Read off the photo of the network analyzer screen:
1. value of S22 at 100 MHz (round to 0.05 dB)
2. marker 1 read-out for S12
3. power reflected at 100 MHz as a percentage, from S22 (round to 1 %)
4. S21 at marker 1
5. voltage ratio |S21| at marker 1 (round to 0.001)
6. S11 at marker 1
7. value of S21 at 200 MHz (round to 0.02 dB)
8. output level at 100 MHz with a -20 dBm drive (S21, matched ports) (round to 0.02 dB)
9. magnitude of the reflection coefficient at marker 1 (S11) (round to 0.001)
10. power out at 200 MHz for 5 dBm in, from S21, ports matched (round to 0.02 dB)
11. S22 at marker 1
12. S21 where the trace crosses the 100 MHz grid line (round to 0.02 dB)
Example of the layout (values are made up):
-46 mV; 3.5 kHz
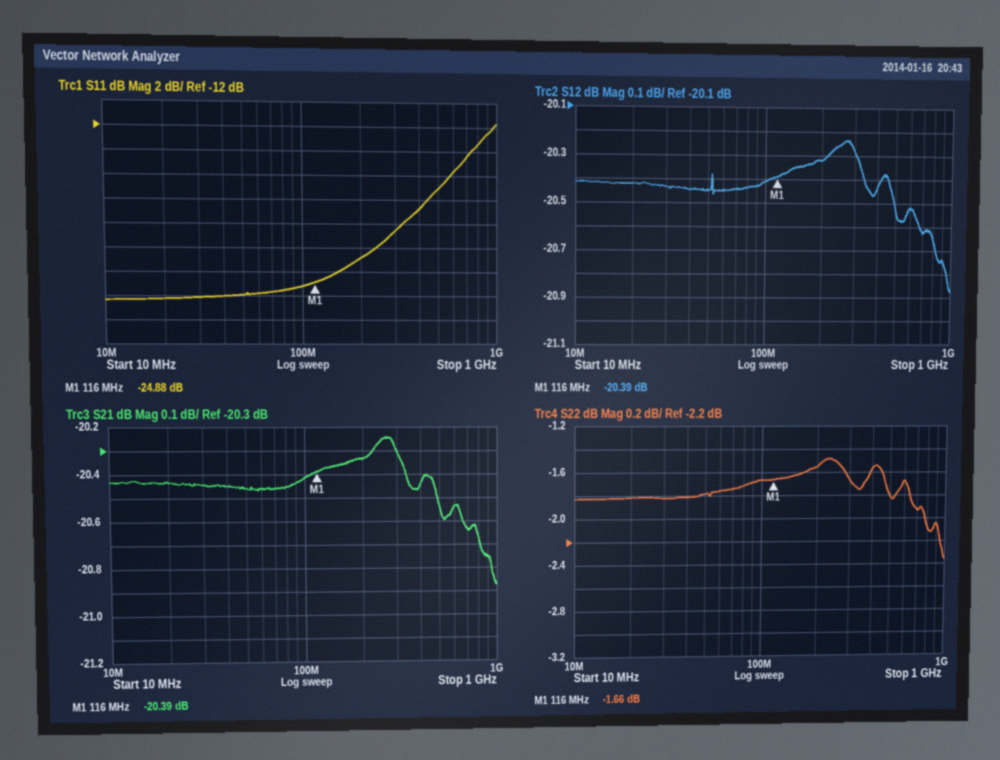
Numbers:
-1.65 dB; -20.39 dB; 68 %; -20.39 dB; 0.096; -24.88 dB; -20.34 dB; -40.42 dBm; 0.057; -15.34 dBm; -1.66 dB; -20.42 dB
